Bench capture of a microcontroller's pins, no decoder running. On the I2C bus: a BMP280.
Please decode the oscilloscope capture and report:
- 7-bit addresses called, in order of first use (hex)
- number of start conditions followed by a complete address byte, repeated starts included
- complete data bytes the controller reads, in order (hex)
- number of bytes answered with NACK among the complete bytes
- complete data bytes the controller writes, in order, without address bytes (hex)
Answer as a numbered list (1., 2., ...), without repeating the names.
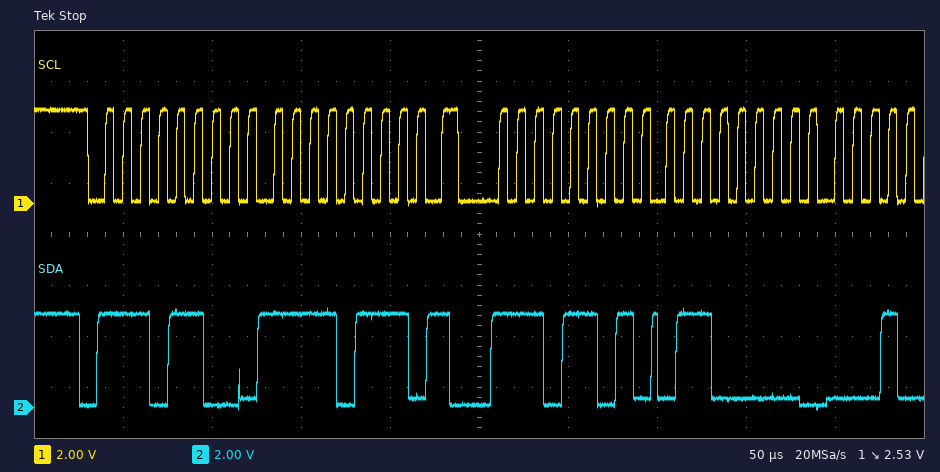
1. 0x76
2. 2
3. 60
4. 0
5. F7
